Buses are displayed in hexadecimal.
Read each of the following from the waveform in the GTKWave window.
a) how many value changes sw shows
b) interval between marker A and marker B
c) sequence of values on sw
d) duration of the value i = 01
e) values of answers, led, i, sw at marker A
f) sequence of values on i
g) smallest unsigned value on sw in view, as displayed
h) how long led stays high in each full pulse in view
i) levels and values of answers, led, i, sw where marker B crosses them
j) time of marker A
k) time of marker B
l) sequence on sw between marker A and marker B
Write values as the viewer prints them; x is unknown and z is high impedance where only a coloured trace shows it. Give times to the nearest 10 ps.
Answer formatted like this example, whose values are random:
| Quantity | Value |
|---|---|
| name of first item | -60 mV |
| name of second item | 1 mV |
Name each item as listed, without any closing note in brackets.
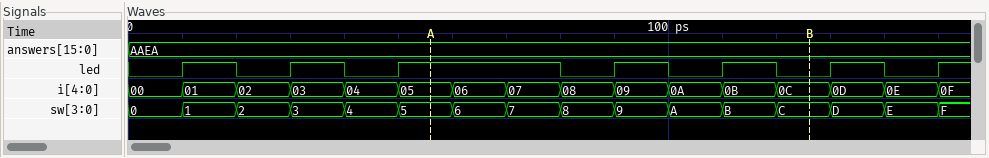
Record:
| Quantity | Value |
|---|---|
| how many value changes sw shows | 15 |
| interval between marker A and marker B | 70 ps |
| sequence of values on sw | 0, 1, 2, 3, 4, 5, 6, 7, 8, 9, A, B, C, D, E, F |
| duration of the value i = 01 | 10 ps |
| values of answers, led, i, sw at marker A | answers=AAEA, led=1, i=05, sw=5 |
| sequence of values on i | 00, 01, 02, 03, 04, 05, 06, 07, 08, 09, 0A, 0B, 0C, 0D, 0E, 0F |
| smallest unsigned value on sw in view, as displayed | 0 |
| how long led stays high in each full pulse in view | 10 ps, 10 ps, 30 ps, 10 ps, 10 ps, 10 ps |
| levels and values of answers, led, i, sw where marker B crosses them | answers=AAEA, led=0, i=0C, sw=C |
| time of marker A | 60 ps |
| time of marker B | 130 ps |
| sequence on sw between marker A and marker B | 5, 6, 7, 8, 9, A, B, C |
